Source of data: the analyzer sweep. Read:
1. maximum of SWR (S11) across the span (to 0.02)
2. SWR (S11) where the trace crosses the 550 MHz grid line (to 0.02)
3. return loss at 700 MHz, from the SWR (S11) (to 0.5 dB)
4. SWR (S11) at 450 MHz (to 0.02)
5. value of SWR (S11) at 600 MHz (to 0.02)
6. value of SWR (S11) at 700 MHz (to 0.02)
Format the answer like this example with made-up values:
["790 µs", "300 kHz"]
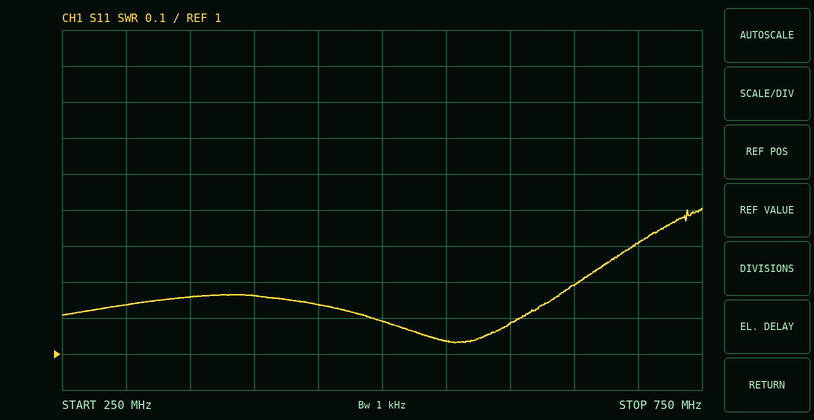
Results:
["1.40", "1.04", "17.5 dB", "1.14", "1.08", "1.30"]
